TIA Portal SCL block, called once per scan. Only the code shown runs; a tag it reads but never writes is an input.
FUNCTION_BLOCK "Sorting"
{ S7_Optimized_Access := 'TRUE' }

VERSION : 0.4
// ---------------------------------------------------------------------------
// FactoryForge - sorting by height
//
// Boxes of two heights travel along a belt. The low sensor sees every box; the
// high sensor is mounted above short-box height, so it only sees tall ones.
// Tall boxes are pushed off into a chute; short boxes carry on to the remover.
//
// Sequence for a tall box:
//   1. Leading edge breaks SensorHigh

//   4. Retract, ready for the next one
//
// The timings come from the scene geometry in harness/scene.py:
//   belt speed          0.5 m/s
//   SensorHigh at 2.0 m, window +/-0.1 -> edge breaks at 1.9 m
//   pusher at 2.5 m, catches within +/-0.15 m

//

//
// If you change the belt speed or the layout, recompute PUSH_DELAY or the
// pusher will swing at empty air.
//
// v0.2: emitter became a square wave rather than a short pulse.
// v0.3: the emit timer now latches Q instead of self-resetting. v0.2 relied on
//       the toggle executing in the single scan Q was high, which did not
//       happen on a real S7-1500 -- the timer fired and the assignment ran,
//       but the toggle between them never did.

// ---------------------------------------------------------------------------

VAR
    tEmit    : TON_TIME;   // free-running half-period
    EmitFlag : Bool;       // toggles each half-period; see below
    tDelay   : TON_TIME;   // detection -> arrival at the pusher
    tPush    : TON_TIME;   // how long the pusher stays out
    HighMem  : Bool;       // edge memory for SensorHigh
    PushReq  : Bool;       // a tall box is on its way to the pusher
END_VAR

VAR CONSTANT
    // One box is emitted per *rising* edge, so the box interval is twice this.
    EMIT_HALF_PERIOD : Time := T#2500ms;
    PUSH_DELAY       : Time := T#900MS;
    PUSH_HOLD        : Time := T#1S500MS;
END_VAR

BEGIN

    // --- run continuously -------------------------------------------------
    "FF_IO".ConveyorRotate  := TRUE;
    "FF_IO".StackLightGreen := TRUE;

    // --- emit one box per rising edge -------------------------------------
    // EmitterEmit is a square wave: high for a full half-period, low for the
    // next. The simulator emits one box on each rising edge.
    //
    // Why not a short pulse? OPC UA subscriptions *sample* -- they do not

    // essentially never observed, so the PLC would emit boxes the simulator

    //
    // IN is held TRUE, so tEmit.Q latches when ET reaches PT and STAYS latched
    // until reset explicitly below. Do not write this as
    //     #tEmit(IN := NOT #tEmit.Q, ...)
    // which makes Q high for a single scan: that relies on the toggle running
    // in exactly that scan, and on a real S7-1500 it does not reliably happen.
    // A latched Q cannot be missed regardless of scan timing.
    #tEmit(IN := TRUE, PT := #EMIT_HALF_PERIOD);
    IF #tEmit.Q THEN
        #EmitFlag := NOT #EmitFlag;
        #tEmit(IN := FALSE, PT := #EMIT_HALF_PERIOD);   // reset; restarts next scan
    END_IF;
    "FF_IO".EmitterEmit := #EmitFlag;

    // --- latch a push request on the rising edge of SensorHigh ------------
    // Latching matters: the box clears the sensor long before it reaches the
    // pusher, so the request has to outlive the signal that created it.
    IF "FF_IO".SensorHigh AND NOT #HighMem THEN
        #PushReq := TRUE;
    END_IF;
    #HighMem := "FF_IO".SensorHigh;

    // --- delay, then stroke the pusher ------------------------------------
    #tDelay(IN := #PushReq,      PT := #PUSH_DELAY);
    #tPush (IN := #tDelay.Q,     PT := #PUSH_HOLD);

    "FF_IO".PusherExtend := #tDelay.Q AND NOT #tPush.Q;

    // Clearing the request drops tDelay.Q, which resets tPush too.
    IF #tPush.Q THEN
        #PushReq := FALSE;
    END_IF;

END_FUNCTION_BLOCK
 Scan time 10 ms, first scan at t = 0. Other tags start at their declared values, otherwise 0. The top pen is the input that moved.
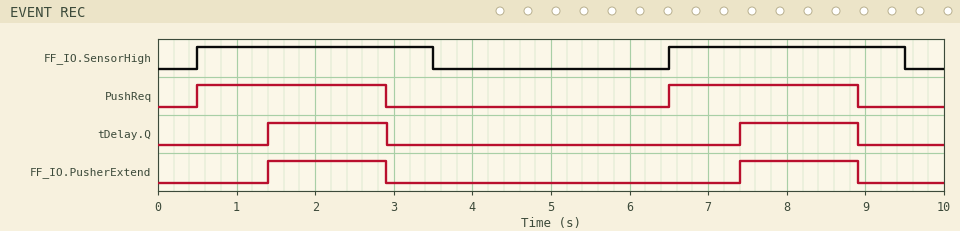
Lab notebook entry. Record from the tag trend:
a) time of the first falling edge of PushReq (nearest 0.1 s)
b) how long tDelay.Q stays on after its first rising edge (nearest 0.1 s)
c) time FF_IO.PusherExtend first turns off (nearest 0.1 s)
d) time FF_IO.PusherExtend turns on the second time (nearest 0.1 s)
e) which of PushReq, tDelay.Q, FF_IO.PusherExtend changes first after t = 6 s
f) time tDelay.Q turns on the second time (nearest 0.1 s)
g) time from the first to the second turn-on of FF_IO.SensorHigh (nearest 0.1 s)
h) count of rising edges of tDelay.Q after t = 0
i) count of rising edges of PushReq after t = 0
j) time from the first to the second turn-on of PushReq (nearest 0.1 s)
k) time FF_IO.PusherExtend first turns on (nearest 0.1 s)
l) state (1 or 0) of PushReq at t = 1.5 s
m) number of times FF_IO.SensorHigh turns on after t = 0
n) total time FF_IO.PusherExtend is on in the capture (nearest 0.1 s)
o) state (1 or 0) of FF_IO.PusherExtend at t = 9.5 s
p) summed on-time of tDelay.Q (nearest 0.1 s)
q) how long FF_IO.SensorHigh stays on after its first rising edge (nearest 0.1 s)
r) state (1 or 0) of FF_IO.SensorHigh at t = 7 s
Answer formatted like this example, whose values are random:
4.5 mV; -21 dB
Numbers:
2.9 s; 1.5 s; 2.9 s; 7.4 s; PushReq; 7.4 s; 6.0 s; 2; 2; 6.0 s; 1.4 s; 1; 2; 3.0 s; 0; 3.0 s; 3.0 s; 1
